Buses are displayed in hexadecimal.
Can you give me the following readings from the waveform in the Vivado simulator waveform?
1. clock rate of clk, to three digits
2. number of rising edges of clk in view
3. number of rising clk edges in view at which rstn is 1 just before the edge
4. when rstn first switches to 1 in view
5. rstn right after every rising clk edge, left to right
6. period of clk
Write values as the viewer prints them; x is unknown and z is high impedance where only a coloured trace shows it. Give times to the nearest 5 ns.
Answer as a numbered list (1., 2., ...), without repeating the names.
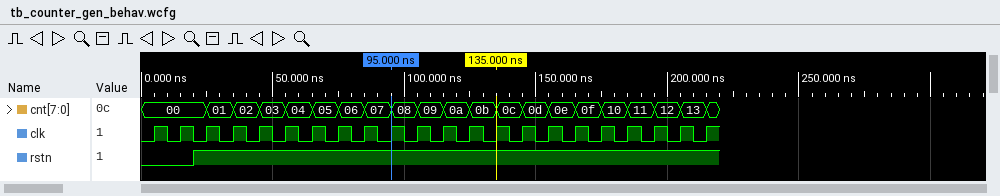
1. 100 MHz
2. 22
3. 20
4. 20 ns
5. 0 0 1 1 1 1 1 1 1 1 1 1 1 1 1 1 1 1 1 1 1 1
6. 10 ns
